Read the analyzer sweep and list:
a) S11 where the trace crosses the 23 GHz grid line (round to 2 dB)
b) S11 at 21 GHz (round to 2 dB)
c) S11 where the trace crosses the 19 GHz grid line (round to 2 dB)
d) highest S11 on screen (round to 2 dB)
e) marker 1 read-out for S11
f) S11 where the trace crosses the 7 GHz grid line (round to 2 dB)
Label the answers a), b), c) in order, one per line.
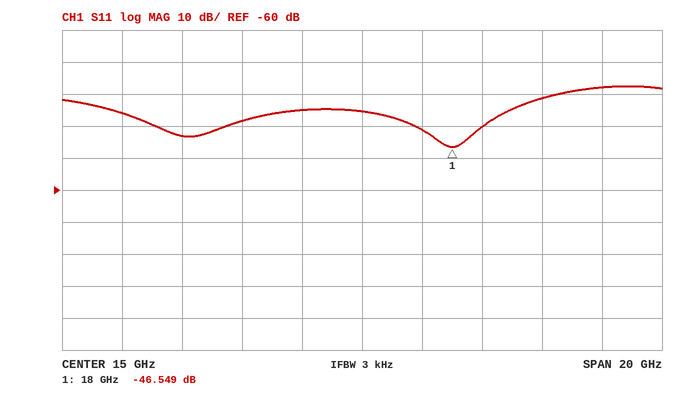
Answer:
a) -28 dB
b) -32 dB
c) -40 dB
d) -28 dB
e) -46.549 dB
f) -36 dB
